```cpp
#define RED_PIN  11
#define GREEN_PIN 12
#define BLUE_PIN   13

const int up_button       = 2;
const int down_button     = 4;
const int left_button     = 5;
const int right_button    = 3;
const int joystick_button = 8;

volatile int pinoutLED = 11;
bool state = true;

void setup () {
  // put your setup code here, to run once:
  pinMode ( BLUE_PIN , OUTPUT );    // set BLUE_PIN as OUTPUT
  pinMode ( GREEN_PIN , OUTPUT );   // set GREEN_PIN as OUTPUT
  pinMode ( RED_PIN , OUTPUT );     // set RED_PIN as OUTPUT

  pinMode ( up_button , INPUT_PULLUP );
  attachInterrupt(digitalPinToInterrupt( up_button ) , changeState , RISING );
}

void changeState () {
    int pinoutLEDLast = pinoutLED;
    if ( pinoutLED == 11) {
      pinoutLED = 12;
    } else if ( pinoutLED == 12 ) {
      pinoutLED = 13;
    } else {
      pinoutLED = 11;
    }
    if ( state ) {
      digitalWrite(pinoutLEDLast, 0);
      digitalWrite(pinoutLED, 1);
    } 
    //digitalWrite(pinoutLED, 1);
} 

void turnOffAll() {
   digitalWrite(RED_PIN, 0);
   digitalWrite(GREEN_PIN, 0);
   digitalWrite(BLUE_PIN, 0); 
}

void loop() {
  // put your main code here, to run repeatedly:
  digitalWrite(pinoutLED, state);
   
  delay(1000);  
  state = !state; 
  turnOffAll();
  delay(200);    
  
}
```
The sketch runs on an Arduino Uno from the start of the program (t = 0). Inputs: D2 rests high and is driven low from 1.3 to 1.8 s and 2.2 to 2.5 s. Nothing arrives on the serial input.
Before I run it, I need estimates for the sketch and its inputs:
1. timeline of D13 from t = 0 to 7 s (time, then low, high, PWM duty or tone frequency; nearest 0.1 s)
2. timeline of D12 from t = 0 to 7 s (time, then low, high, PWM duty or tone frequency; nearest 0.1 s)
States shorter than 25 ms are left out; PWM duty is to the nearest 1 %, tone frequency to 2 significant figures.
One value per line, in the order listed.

0 s low; 2.5 s high; 3.4 s low; 4.8 s high; 5.8 s low
0 s low; 2.4 s high; 2.5 s low
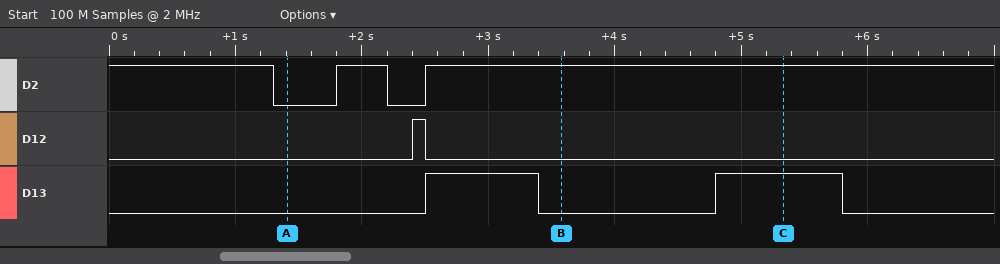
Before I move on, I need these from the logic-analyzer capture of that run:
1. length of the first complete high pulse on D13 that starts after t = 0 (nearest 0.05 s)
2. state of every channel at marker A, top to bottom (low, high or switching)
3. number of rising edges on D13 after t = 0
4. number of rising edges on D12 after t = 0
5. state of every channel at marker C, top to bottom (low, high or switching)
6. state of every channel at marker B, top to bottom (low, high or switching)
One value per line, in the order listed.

0.90 s
D2 low, D12 low, D13 low
2
1
D2 high, D12 low, D13 high
D2 high, D12 low, D13 low
